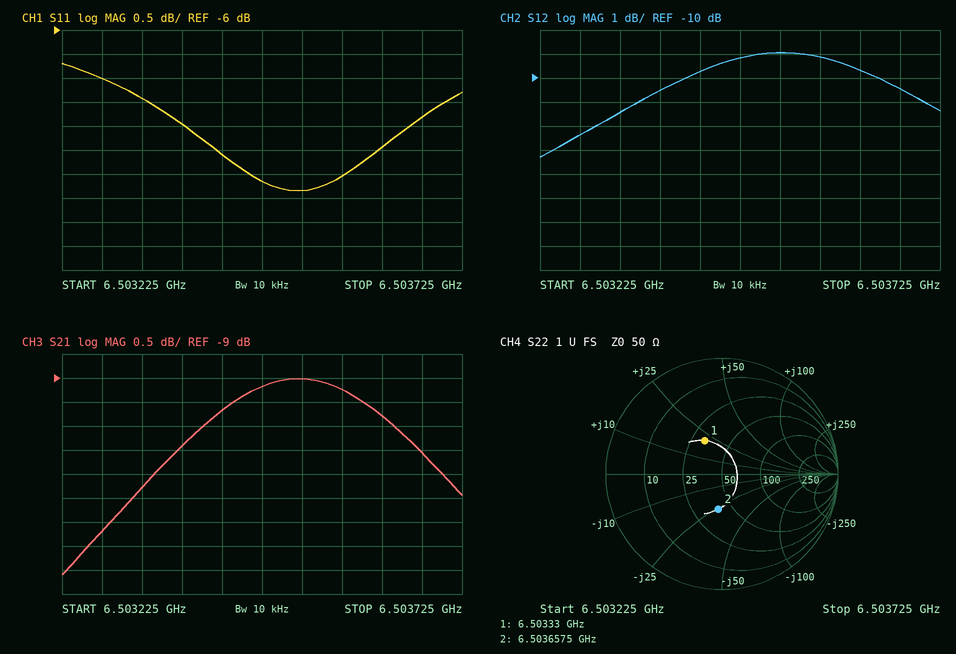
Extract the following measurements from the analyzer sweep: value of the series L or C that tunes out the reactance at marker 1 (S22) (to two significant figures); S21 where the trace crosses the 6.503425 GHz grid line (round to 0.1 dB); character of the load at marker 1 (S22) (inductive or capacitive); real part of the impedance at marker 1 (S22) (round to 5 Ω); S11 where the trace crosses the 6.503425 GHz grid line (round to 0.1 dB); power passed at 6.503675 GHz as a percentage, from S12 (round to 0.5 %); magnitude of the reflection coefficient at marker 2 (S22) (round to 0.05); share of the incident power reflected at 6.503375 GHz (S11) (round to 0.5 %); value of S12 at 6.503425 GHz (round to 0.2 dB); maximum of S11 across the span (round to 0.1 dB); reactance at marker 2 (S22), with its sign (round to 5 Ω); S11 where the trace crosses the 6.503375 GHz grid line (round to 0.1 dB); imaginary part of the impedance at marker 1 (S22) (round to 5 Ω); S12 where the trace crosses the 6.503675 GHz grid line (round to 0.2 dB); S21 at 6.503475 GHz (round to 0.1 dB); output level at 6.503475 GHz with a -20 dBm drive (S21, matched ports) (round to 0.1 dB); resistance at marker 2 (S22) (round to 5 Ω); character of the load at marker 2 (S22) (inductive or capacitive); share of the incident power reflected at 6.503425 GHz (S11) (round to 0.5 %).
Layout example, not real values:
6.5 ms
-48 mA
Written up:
1.2 pF
-9.7 dB
inductive
30 Ω
-8.6 dB
9.0 %
0.30
16.0 %
-9.8 dB
-6.7 dB
-25 Ω
-8.0 dB
+20 Ω
-10.4 dB
-9.2 dB
-29.2 dBm
40 Ω
capacitive
14.0 %
